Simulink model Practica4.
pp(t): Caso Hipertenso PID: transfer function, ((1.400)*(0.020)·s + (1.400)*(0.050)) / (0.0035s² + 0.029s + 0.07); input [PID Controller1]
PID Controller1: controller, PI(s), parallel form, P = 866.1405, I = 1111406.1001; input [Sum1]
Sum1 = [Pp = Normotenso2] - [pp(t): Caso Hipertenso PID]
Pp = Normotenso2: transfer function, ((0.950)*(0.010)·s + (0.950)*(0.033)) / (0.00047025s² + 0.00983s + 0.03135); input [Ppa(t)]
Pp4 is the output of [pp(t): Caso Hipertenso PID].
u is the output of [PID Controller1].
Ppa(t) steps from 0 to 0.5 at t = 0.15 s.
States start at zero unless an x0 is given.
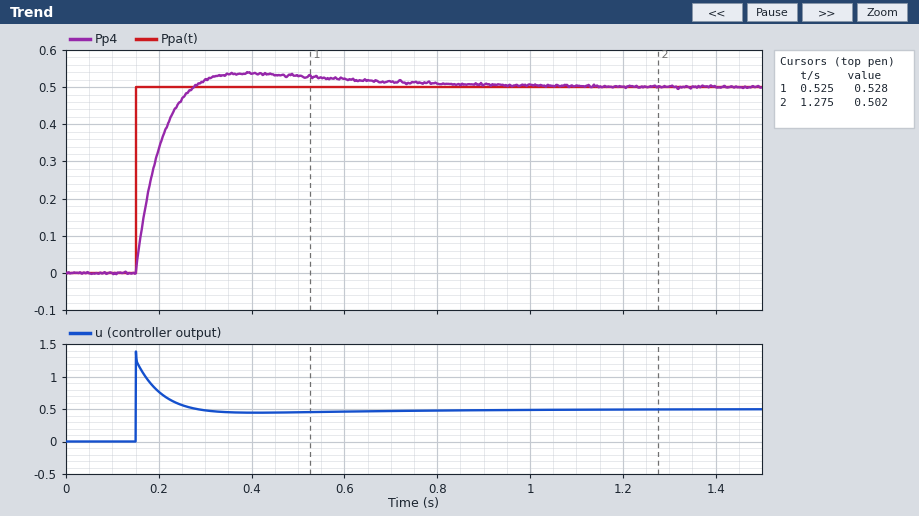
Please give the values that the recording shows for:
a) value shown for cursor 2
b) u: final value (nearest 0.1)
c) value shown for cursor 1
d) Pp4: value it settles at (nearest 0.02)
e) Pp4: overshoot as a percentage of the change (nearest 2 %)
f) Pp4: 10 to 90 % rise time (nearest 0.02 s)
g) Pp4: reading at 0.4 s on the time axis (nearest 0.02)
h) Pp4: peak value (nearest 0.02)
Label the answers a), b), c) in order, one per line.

a) 0.502
b) 0.5
c) 0.528
d) 0.50
e) 8 %
f) 0.08 s
g) 0.54
h) 0.54
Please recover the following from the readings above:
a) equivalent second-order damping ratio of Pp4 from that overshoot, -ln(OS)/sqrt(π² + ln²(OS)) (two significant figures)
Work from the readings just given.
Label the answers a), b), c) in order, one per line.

a) 0.63
